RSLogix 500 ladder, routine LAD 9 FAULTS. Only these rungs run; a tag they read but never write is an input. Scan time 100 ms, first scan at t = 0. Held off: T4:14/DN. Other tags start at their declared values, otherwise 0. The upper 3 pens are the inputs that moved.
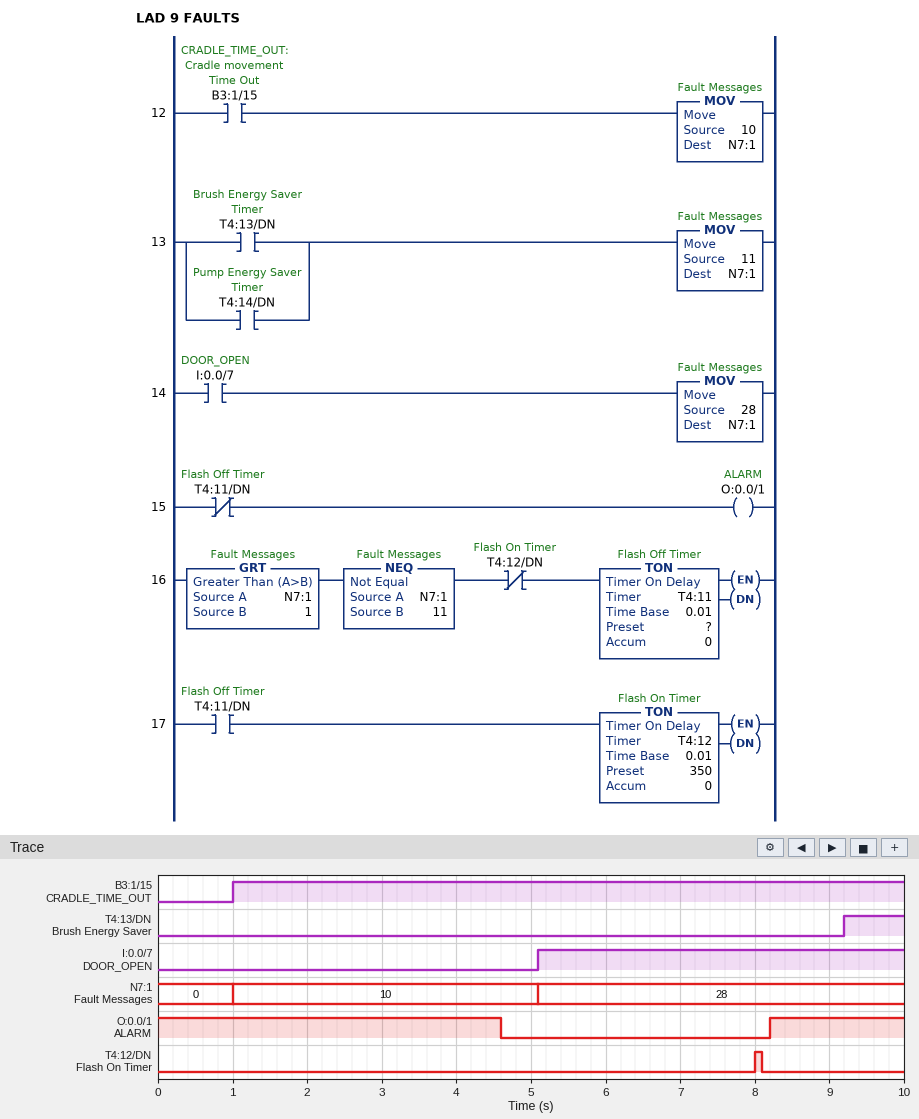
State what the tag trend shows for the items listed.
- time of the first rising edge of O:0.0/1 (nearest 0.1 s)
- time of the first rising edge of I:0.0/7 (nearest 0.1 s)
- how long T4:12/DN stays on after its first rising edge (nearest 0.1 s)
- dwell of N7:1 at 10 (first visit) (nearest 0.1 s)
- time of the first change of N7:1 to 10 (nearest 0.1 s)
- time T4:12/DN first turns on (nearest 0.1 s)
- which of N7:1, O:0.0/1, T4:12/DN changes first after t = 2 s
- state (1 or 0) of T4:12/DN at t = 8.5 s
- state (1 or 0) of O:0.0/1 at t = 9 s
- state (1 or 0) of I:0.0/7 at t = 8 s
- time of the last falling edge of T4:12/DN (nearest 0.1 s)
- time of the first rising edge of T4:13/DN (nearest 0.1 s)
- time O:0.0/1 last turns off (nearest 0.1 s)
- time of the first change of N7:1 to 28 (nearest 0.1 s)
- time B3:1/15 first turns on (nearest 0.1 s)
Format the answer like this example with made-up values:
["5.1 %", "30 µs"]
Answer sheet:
["8.2 s", "5.1 s", "0.1 s", "4.1 s", "1.0 s", "8.0 s", "O:0.0/1", "0", "1", "1", "8.1 s", "9.2 s", "4.6 s", "5.1 s", "1.0 s"]
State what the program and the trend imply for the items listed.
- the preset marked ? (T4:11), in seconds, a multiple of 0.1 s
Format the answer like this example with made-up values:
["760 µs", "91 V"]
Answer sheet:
["3.5 s"]
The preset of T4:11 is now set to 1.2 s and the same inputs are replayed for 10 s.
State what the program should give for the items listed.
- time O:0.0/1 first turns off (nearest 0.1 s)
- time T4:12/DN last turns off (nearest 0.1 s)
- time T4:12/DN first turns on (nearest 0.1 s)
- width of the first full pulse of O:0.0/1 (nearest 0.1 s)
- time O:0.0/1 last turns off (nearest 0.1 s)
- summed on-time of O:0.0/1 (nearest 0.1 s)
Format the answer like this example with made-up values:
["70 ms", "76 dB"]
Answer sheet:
["2.3 s", "5.8 s", "5.7 s", "1.3 s", "7.2 s", "3.6 s"]
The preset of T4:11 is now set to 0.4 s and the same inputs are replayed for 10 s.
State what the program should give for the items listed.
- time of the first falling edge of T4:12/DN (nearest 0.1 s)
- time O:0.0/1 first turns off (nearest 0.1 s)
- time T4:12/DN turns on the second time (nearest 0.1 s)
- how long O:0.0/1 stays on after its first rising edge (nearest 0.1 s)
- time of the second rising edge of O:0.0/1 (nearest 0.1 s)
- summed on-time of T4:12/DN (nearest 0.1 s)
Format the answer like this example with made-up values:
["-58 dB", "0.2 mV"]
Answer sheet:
["5.0 s", "1.5 s", "9.0 s", "0.5 s", "9.2 s", "0.2 s"]
